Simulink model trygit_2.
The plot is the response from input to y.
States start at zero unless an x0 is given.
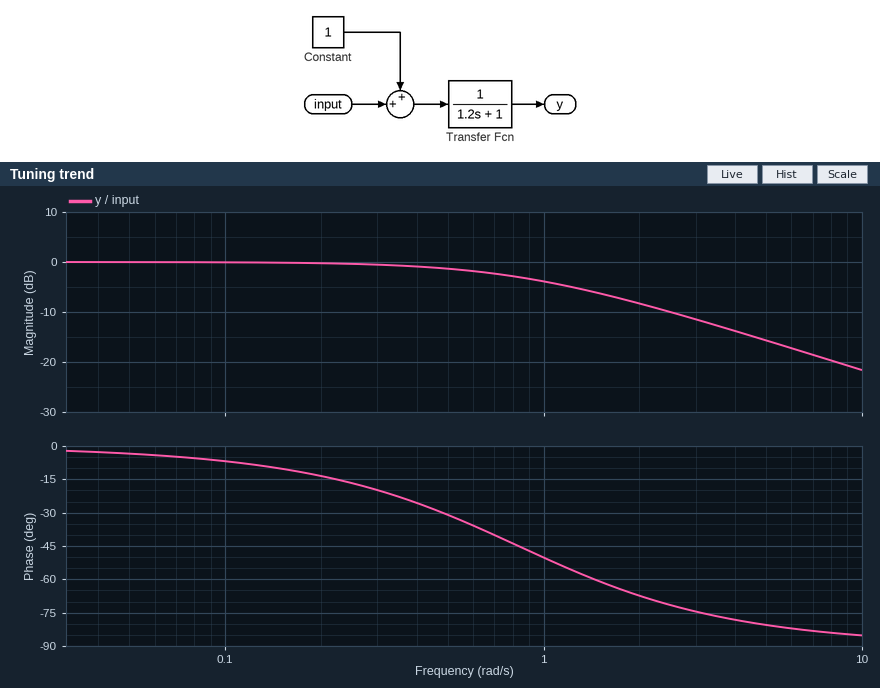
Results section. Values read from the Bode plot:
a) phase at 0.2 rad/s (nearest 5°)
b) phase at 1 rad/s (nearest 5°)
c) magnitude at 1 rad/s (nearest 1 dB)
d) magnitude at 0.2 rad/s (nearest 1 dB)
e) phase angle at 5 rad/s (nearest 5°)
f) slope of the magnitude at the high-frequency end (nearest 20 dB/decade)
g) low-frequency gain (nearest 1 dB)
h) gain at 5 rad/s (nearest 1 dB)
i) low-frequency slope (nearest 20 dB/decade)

-15°
-50°
-4 dB
0 dB
-80°
-20 dB/decade
0 dB
-16 dB
0 dB/decade
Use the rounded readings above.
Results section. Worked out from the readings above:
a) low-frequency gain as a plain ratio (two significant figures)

1.0
